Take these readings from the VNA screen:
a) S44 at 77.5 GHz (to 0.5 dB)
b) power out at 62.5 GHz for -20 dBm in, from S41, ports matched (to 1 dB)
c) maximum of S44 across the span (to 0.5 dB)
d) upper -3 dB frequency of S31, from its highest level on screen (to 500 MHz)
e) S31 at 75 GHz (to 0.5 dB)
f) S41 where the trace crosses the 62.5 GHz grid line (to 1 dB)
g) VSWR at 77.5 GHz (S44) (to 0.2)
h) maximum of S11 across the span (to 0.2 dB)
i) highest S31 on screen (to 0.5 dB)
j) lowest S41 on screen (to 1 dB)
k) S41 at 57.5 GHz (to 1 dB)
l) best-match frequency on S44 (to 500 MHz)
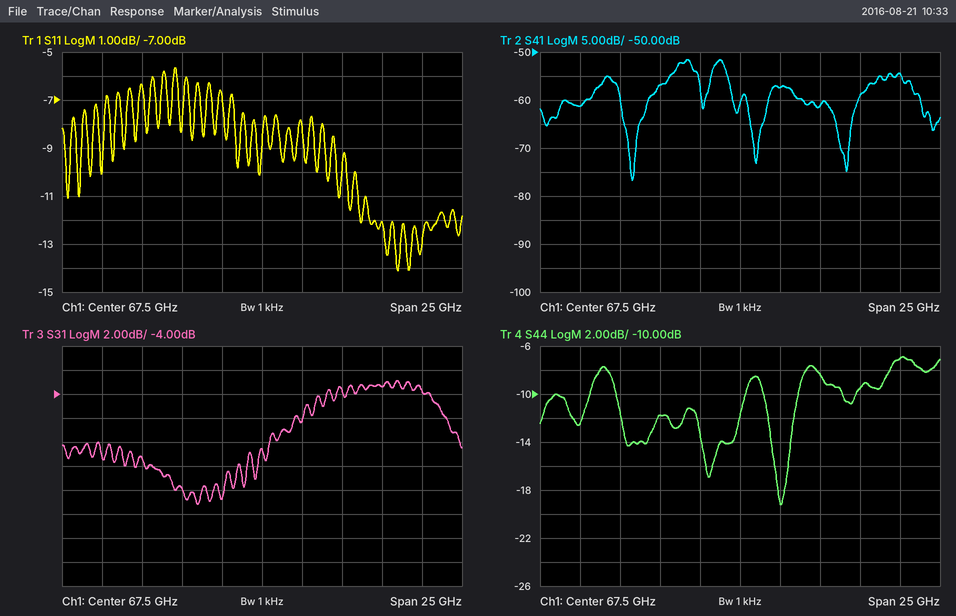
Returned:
-7.0 dB
-77 dBm
-7.0 dB
79.0 GHz
-3.5 dB
-57 dB
2.6
-5.6 dB
-3.0 dB
-77 dB
-61 dB
70.0 GHz
